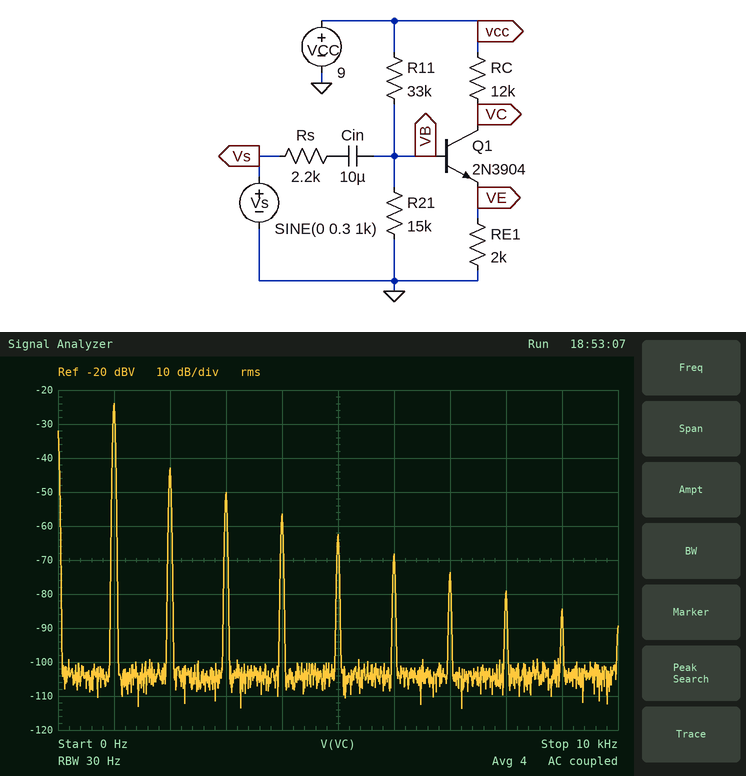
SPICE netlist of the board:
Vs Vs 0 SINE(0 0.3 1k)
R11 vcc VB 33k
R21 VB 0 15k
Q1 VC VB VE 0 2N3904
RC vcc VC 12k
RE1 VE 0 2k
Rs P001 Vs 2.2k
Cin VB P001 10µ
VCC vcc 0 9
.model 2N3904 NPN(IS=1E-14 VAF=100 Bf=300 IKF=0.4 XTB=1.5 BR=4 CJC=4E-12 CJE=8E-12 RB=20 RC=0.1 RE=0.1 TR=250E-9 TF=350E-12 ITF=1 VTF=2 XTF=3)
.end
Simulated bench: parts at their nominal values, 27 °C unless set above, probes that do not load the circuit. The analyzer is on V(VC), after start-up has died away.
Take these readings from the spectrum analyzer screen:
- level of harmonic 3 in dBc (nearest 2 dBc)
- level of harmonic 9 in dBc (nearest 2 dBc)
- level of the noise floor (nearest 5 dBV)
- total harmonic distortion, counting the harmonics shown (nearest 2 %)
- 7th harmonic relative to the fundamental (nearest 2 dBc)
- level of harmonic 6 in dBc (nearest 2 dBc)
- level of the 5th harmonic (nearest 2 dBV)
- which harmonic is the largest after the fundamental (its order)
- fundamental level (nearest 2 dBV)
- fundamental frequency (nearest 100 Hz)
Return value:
-26 dBc
-60 dBc
-105 dBV
12 %
-50 dBc
-44 dBc
-62 dBV
2
-24 dBV
1.0 kHz
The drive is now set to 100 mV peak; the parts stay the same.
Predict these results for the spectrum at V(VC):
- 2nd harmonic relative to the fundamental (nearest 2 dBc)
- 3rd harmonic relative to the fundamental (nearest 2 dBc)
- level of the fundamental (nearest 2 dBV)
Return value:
-36 dBc
-54 dBc
-32 dBV
